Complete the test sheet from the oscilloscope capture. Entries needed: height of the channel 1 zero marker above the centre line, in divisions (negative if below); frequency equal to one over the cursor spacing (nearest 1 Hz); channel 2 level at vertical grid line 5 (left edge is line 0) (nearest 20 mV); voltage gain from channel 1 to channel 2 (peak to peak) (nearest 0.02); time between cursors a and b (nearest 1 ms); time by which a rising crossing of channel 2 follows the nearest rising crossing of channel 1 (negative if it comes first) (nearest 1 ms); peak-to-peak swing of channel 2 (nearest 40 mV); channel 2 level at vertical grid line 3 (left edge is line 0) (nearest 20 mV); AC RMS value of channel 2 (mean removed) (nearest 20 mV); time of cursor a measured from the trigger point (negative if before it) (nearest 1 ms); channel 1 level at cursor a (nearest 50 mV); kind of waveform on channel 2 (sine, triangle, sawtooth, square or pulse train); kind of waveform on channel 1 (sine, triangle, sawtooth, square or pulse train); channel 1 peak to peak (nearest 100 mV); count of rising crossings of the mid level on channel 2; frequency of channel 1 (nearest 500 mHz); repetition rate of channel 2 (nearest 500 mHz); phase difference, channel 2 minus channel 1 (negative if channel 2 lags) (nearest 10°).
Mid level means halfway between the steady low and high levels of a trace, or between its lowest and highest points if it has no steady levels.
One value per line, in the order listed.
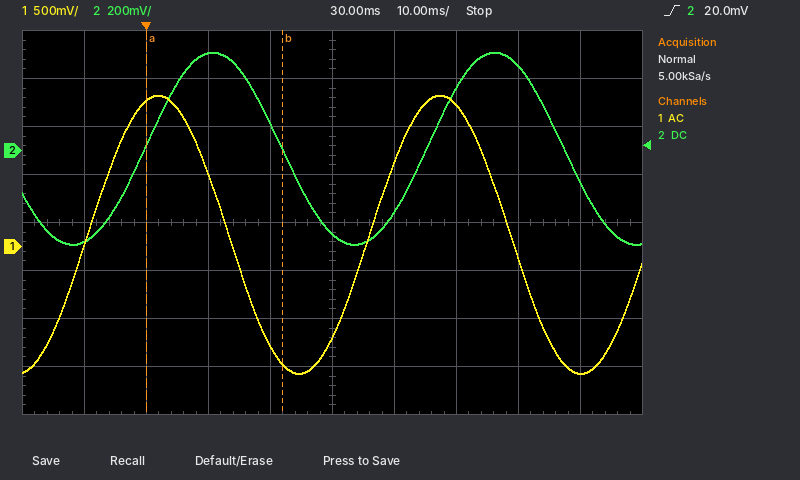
-0.5 div
45 Hz
-340 mV
0.28
22 ms
+9 ms
800 mV
400 mV
280 mV
0 ms
1.50 V
sine
sine
2.90 V
2
22.0 Hz
22.0 Hz
-70°
